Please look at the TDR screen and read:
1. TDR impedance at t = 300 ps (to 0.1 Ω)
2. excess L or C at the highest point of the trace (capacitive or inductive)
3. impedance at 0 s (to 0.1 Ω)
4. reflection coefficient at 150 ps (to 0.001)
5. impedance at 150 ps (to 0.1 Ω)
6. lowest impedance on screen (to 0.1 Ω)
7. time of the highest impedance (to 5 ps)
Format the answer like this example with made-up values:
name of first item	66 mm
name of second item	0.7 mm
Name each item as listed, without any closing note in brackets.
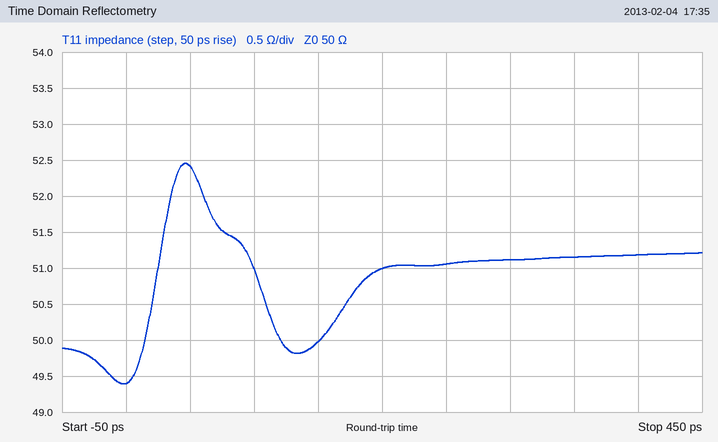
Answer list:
TDR impedance at t = 300 ps	51.1 Ω
excess L or C at the highest point of the trace	inductive
impedance at 0 s	49.4 Ω
reflection coefficient at 150 ps	0.000
impedance at 150 ps	50.0 Ω
lowest impedance on screen	49.4 Ω
time of the highest impedance	45 ps
